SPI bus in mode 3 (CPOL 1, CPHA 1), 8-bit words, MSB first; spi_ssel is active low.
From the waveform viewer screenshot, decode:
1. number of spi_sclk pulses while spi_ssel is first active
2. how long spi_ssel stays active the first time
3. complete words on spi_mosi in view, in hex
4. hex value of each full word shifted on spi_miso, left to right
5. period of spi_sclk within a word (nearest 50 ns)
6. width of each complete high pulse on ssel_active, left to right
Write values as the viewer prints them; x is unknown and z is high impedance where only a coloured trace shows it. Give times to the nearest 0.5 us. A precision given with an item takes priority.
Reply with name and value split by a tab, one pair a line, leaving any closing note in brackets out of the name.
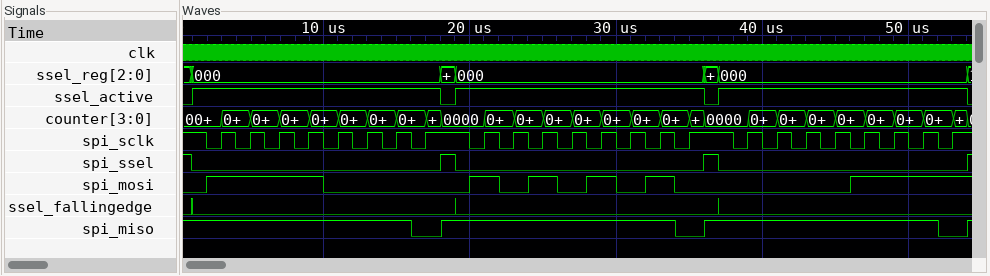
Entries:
number of spi_sclk pulses while spi_ssel is first active	8
how long spi_ssel stays active the first time	17 us
complete words on spi_mosi in view, in hex	F0, AA, 0F
hex value of each full word shifted on spi_miso, left to right	FE, FE, FE
period of spi_sclk within a word	2000 ns
width of each complete high pulse on ssel_active, left to right	17 us, 17 us, 17 us
